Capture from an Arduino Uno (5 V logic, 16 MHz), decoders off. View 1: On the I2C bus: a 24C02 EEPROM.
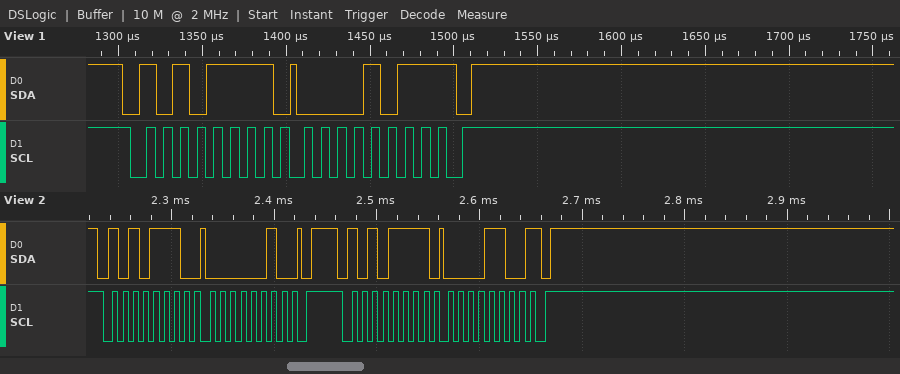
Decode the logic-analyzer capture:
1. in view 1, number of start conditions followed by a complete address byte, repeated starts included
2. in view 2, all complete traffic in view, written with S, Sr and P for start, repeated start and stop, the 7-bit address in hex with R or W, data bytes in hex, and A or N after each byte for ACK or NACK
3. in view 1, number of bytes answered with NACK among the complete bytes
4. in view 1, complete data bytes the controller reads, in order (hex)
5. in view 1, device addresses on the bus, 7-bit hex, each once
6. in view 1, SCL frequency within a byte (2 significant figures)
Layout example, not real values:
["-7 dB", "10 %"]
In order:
["1", "S 57W A 02 A P S 57R A 0C N P", "1", "0B", "0x57", "100 kHz"]
